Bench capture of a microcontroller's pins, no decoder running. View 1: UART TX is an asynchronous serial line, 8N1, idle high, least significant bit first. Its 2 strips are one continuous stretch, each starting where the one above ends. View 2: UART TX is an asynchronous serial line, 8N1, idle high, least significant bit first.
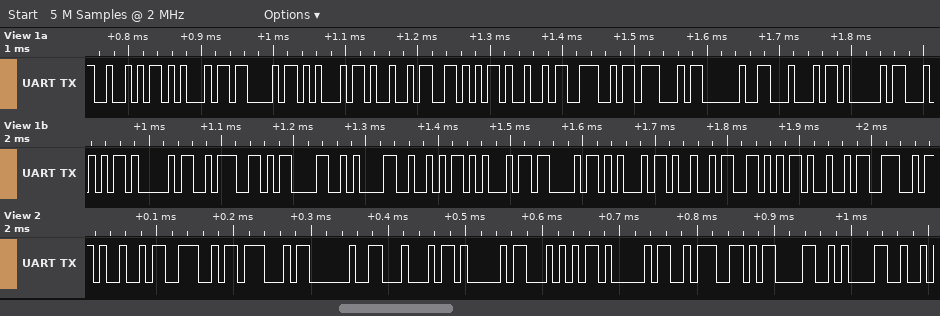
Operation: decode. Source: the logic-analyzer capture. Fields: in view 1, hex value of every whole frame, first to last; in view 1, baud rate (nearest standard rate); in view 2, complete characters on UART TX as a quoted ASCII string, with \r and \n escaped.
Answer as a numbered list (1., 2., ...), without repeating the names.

1. 0x52 0x45 0x43 0x45 0x49 0x56 0x49 0x4E 0x47 0x20 0x44 0x41 0x54 0x41 0x3A 0x0D 0x0A 0x52 0x45 0x43 0x45 0x49 0x56 0x49 0x4E
2. 115200 baud
3. "ING DATA:\r\n"
